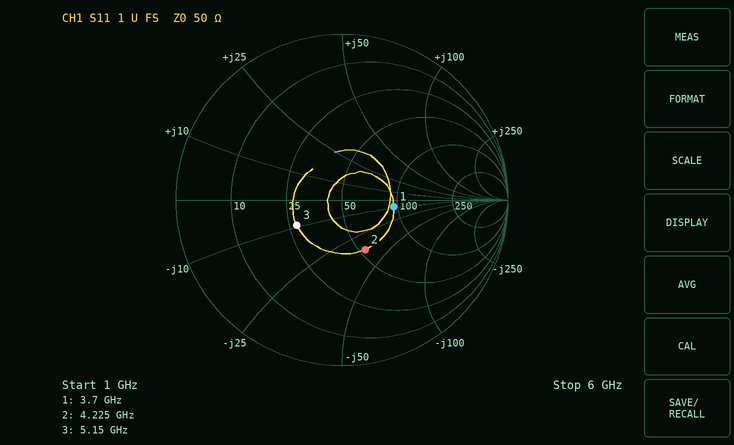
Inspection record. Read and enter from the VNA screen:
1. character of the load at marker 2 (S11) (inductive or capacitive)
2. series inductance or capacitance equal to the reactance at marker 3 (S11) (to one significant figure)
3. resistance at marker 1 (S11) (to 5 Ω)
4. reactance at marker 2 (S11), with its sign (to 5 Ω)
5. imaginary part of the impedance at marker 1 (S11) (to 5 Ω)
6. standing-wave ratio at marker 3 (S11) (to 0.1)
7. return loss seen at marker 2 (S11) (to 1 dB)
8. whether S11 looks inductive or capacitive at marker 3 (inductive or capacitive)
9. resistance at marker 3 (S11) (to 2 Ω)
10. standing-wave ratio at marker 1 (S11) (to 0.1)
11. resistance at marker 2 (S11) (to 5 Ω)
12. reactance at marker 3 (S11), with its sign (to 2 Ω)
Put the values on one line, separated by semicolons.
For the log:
capacitive; 3 pF; 95 Ω; -35 Ω; -10 Ω; 1.9; 10 dB; capacitive; 28 Ω; 1.9; 55 Ω; -10 Ω
